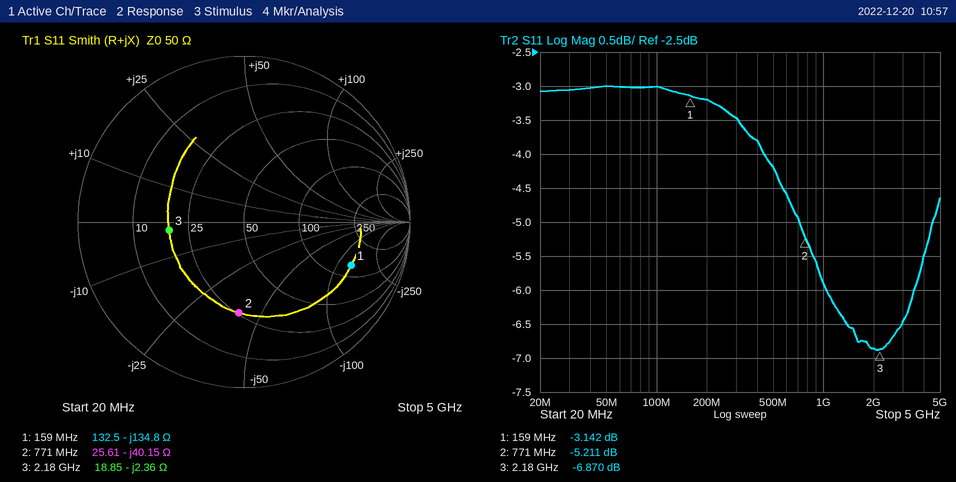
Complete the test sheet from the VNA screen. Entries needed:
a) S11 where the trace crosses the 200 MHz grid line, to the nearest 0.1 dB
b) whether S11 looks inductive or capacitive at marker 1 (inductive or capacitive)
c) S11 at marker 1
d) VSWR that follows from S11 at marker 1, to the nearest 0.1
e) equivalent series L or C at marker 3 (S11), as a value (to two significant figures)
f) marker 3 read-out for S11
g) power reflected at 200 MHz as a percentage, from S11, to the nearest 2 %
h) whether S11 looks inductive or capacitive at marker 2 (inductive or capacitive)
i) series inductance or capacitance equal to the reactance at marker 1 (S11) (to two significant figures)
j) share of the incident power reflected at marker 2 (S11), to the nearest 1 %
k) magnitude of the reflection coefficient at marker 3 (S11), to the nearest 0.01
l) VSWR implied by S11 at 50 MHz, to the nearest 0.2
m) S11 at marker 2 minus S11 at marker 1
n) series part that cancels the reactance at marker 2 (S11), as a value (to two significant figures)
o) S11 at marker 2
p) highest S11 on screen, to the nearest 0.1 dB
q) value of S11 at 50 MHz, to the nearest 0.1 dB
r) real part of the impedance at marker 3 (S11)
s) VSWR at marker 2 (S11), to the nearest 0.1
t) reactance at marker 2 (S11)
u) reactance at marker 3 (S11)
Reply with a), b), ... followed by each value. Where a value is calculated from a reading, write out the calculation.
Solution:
a) -3.2 dB
b) capacitive
c) -3.142 dB
d) (1 + 0.6965)/(1 − 0.6965) ≈ 5.6
e) C = 1/(2π × 2.18 GHz × 2.36 Ω) ≈ 31 pF
f) -6.870 dB
g) 10^(-3.2/10) ≈ 48 %
h) capacitive
i) C = 1/(2π × 159 MHz × 134.8 Ω) ≈ 7.4 pF
j) 10^(-5.211/10) ≈ 30 %
k) 0.45
l) |Γ| = 10^(-3/20) = 0.7079; VSWR = (1 + 0.7079)/(1 − 0.7079) ≈ 5.8
m) -5.211 − (-3.142) = -2.069 dB
n) L = 40.15 Ω/(2π × 771 MHz) ≈ 8.3 nH
o) -5.211 dB
p) -3.0 dB
q) -3.0 dB
r) 18.85 Ω
s) 3.4
t) -40.15 Ω
u) -2.36 Ω
